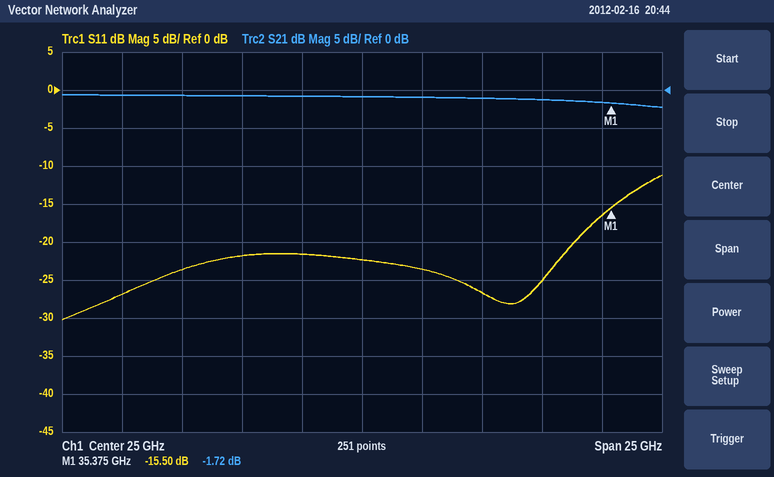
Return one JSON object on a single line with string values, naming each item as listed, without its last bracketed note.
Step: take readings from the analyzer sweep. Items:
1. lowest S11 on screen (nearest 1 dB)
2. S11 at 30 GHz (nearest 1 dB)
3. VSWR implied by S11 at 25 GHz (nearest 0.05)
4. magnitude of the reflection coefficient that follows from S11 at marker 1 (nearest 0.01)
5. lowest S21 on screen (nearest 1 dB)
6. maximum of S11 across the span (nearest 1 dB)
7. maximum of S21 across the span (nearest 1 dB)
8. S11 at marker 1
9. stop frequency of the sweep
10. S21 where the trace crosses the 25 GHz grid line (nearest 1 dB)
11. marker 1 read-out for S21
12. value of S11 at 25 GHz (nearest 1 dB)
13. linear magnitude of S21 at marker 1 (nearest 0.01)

{"lowest S11 on screen": "-30 dB", "S11 at 30 GHz": "-27 dB", "VSWR implied by S11 at 25 GHz": "1.15", "magnitude of the reflection coefficient that follows from S11 at marker 1": "0.17", "lowest S21 on screen": "-2 dB", "maximum of S11 across the span": "-11 dB", "maximum of S21 across the span": "-1 dB", "S11 at marker 1": "-15.50 dB", "stop frequency of the sweep": "37.5 GHz", "S21 where the trace crosses the 25 GHz grid line": "-1 dB", "marker 1 read-out for S21": "-1.72 dB", "value of S11 at 25 GHz": "-22 dB", "linear magnitude of S21 at marker 1": "0.82"}
